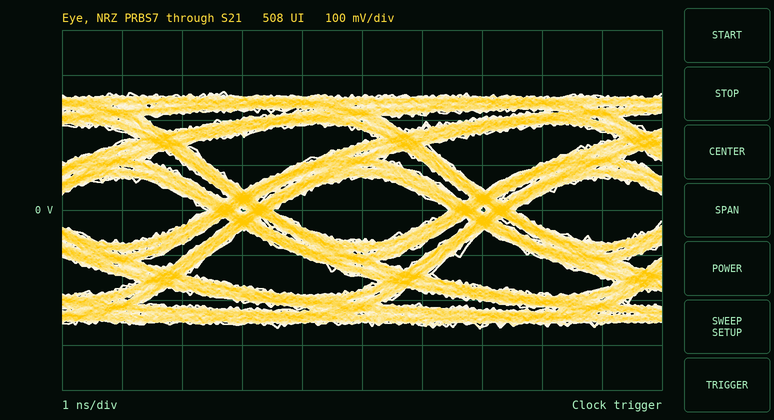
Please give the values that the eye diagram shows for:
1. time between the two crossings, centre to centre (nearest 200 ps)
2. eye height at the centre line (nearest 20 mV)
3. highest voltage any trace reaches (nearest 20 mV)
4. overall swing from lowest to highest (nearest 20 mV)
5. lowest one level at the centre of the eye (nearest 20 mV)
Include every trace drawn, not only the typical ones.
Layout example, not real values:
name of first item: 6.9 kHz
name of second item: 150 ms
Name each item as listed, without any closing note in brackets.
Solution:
time between the two crossings, centre to centre: 4.0 ns
eye height at the centre line: 140 mV
highest voltage any trace reaches: 260 mV
overall swing from lowest to highest: 520 mV
lowest one level at the centre of the eye: 80 mV
